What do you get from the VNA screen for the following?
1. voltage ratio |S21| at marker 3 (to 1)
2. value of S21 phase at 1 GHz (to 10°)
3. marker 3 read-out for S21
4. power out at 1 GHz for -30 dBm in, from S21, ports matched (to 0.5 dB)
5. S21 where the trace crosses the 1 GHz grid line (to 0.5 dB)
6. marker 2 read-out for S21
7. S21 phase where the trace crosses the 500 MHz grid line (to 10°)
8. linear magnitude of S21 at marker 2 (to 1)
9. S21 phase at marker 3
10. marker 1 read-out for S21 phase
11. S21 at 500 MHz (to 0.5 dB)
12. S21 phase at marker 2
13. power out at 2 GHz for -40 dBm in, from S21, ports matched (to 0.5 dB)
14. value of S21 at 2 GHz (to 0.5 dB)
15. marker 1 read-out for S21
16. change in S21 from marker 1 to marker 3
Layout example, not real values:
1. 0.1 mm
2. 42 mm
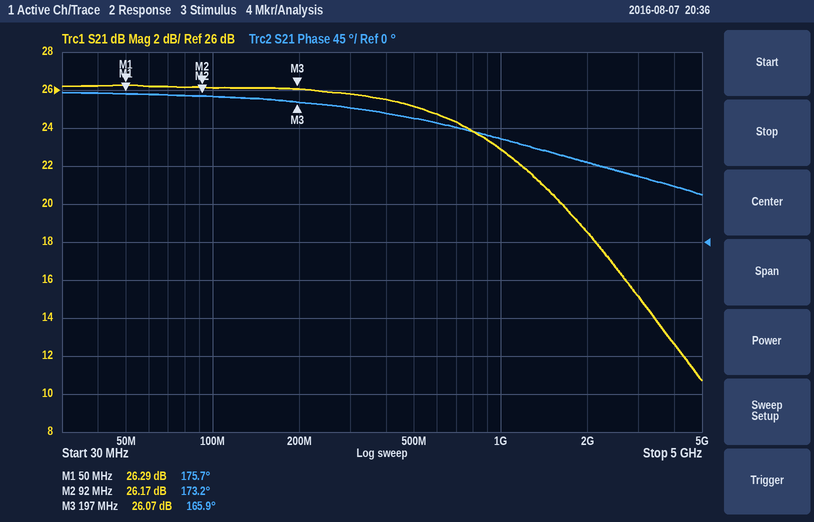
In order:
1. 20
2. 120°
3. 26.07 dB
4. -7.0 dBm
5. 23.0 dB
6. 26.17 dB
7. 150°
8. 20
9. 165.9°
10. 175.7°
11. 25.0 dB
12. 173.2°
13. -21.5 dBm
14. 18.5 dB
15. 26.29 dB
16. -0.22 dB
